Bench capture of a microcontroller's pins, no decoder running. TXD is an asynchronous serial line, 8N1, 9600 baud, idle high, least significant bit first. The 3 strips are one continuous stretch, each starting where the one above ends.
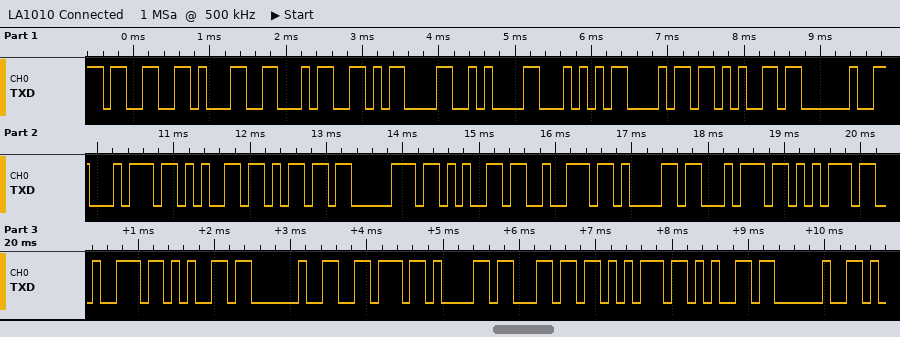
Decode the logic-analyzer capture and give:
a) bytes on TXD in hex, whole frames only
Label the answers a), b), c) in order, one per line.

a) 33 31 34 0D 0A 54 68 65 20 74 65 6D 70 65 72 61 74 75 72 65 20 76 61 6C 75 65 20
